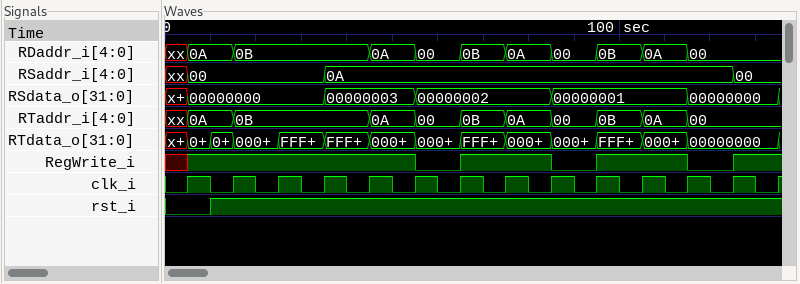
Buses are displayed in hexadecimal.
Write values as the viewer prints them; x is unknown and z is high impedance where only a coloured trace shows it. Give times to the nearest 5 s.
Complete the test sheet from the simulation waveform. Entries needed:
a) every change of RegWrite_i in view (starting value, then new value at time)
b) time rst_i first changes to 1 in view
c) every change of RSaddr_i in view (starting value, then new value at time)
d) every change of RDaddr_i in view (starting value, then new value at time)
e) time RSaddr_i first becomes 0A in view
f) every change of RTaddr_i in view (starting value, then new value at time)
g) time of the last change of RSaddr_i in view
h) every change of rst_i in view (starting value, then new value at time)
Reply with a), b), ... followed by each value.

a) x, 1 at 5 s, 0 at 55 s, 1 at 65 s, 0 at 85 s, 1 at 95 s, 0 at 115 s, 1 at 125 s
b) 10 s
c) xx, 00 at 5 s, 0A at 35 s, 00 at 125 s
d) xx, 0A at 5 s, 0B at 15 s, 0A at 45 s, 00 at 55 s, 0B at 65 s, 0A at 75 s, 00 at 85 s, 0B at 95 s, 0A at 105 s, 00 at 115 s
e) 35 s
f) xx, 0A at 5 s, 0B at 15 s, 0A at 45 s, 00 at 55 s, 0B at 65 s, 0A at 75 s, 00 at 85 s, 0B at 95 s, 0A at 105 s, 00 at 115 s
g) 125 s
h) 0, 1 at 10 s
